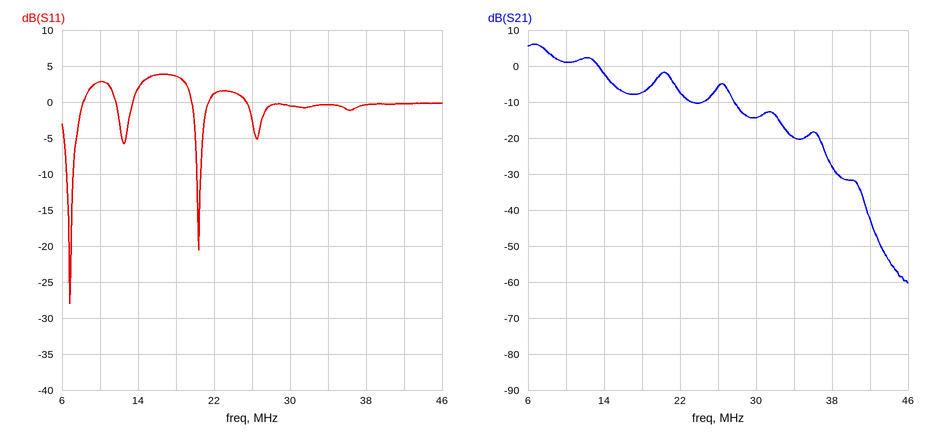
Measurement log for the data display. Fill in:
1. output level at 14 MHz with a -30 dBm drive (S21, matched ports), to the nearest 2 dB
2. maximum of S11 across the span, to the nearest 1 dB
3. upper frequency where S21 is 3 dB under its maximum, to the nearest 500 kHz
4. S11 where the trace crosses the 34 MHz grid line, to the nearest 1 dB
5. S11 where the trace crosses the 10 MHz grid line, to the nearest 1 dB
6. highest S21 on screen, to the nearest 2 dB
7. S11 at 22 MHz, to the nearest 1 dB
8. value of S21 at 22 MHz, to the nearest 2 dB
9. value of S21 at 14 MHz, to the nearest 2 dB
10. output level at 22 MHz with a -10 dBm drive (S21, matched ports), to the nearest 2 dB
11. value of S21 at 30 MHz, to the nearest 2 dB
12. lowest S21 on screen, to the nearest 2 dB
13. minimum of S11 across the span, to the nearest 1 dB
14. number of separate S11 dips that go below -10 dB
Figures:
-32 dBm
4 dB
8.5 MHz
0 dB
3 dB
6 dB
1 dB
-8 dB
-2 dB
-18 dBm
-14 dB
-60 dB
-28 dB
2
